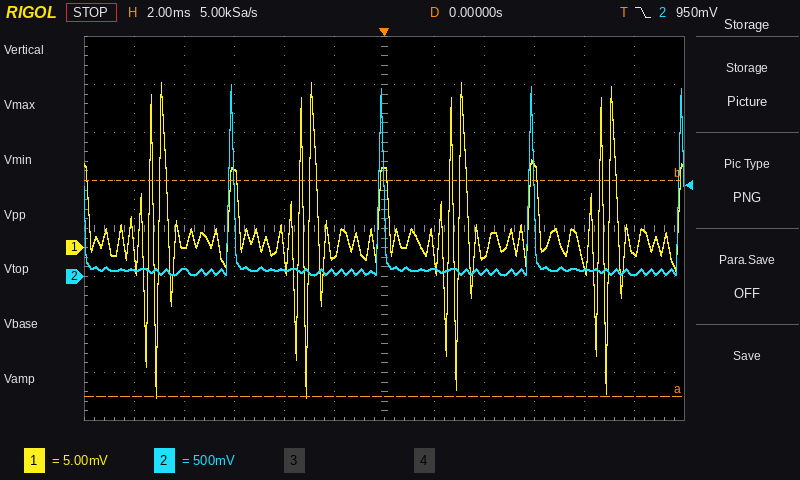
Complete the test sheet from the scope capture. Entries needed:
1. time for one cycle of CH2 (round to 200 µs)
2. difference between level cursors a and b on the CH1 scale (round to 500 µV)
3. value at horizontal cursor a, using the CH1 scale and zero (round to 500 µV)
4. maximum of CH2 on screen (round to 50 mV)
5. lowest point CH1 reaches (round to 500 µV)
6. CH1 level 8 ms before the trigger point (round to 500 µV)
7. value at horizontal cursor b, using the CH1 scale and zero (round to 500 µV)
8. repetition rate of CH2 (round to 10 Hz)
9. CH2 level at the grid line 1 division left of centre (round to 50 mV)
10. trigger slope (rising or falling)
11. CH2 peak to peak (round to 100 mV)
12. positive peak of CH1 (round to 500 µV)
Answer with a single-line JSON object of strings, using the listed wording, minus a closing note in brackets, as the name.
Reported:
{"time for one cycle of CH2": "6.0 ms", "difference between level cursors a and b on the CH1 scale": "22.5 mV", "value at horizontal cursor a, using the CH1 scale and zero": "-15.5 mV", "maximum of CH2 on screen": "2.00 V", "lowest point CH1 reaches": "-15.5 mV", "CH1 level 8 ms before the trigger point": "0.0 mV", "value at horizontal cursor b, using the CH1 scale and zero": "7.0 mV", "repetition rate of CH2": "170 Hz", "CH2 level at the grid line 1 division left of centre": "50 mV", "trigger slope": "falling", "CH2 peak to peak": "2.00 V", "positive peak of CH1": "17.0 mV"}
